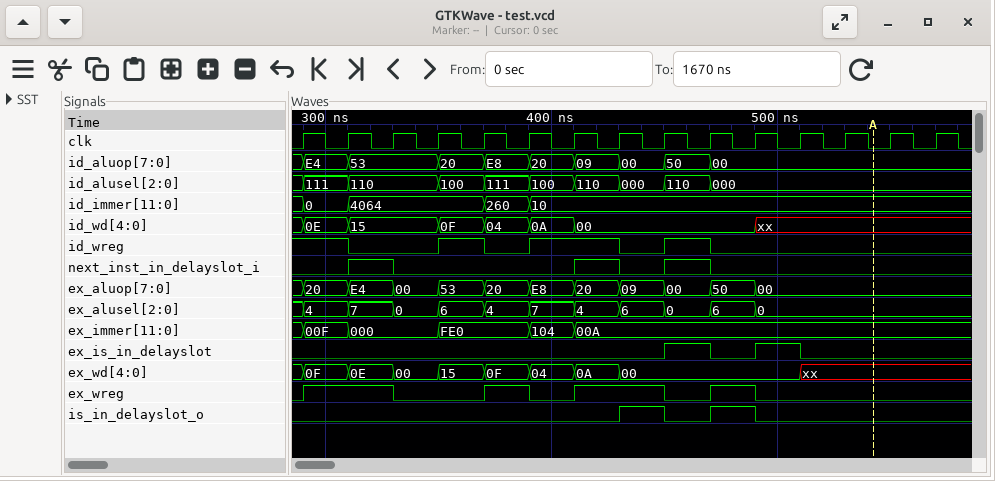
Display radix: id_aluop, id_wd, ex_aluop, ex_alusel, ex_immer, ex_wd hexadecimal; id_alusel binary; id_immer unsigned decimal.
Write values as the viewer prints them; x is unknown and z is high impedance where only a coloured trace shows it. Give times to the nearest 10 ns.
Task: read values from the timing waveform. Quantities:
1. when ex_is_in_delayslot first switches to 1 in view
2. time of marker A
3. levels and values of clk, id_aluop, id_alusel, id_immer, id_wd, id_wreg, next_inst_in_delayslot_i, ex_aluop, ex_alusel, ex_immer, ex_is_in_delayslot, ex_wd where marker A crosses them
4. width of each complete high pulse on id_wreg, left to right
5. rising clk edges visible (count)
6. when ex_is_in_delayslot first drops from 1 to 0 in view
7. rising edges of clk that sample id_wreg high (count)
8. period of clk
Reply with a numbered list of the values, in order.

1. 450 ns
2. 540 ns
3. clk=0, id_aluop=00, id_alusel=000, id_immer=10, id_wd=xx, id_wreg=0, next_inst_in_delayslot_i=0, ex_aluop=00, ex_alusel=0, ex_immer=00A, ex_is_in_delayslot=0, ex_wd=xx
4. 20 ns, 40 ns, 20 ns
5. 15
6. 470 ns
7. 6
8. 20 ns
